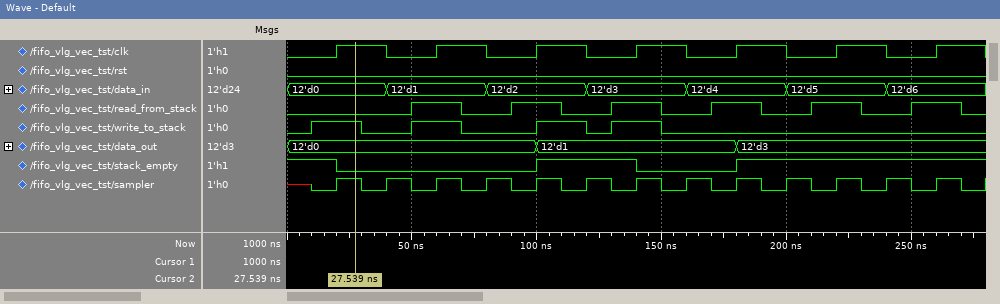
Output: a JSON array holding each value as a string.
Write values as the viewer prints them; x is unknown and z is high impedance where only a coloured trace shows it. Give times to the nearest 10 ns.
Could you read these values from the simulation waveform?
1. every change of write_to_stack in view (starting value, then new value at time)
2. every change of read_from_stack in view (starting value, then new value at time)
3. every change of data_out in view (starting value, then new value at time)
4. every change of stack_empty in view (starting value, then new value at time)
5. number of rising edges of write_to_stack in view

["0, 1 at 10 ns, 0 at 30 ns, 1 at 50 ns, 0 at 70 ns, 1 at 100 ns, 0 at 120 ns, 1 at 130 ns, 0 at 150 ns", "0, 1 at 50 ns, 0 at 70 ns, 1 at 90 ns, 0 at 110 ns, 1 at 130 ns, 0 at 150 ns, 1 at 170 ns, 0 at 190 ns, 1 at 210 ns, 0 at 230 ns, 1 at 250 ns, 0 at 270 ns", "12'd0, 12'd1 at 100 ns, 12'd3 at 180 ns", "1, 0 at 20 ns, 1 at 100 ns, 0 at 140 ns, 1 at 180 ns", "4"]
